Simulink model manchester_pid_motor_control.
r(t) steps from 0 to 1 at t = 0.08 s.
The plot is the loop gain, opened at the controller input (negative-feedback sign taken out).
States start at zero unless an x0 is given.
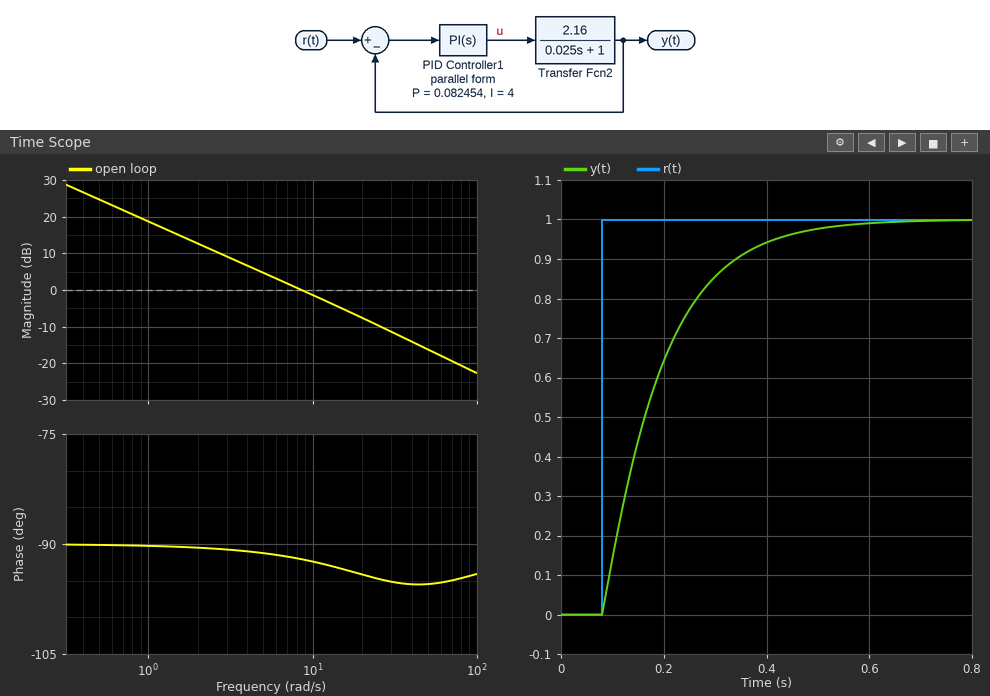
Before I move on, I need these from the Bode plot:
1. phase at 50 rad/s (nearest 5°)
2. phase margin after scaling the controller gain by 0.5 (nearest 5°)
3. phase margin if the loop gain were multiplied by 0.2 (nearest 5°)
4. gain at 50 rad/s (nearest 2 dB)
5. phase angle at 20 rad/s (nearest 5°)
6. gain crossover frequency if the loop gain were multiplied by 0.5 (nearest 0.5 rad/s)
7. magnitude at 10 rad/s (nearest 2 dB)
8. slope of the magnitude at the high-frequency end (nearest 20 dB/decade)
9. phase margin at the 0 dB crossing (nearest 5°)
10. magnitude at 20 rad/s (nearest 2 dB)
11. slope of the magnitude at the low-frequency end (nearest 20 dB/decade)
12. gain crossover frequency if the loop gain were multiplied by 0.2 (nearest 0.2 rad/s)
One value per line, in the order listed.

-95°
90°
90°
-16 dB
-95°
4.5 rad/s
-2 dB
-20 dB/decade
90°
-8 dB
-20 dB/decade
1.8 rad/s
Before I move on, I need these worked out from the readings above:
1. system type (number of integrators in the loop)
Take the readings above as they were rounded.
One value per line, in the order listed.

1
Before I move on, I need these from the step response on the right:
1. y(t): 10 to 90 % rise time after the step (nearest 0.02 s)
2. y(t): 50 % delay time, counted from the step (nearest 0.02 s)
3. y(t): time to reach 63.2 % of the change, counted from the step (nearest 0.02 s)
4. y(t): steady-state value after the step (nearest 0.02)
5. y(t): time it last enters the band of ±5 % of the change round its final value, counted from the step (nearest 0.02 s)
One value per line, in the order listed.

0.24 s
0.08 s
0.12 s
1.00
0.34 s
